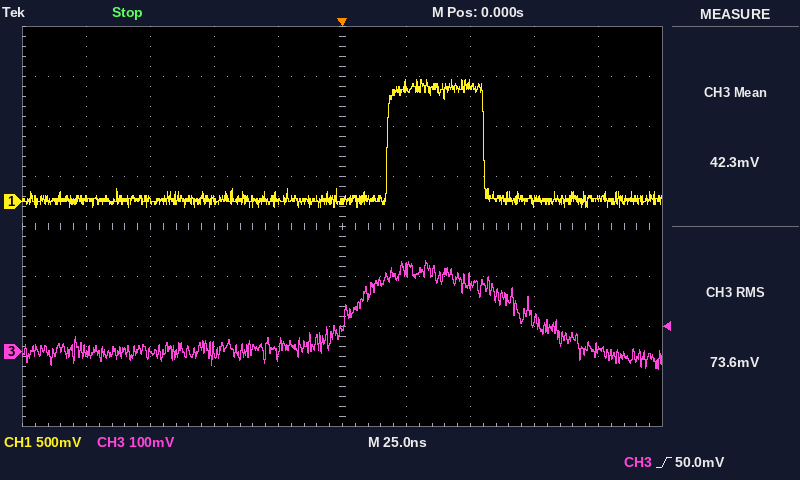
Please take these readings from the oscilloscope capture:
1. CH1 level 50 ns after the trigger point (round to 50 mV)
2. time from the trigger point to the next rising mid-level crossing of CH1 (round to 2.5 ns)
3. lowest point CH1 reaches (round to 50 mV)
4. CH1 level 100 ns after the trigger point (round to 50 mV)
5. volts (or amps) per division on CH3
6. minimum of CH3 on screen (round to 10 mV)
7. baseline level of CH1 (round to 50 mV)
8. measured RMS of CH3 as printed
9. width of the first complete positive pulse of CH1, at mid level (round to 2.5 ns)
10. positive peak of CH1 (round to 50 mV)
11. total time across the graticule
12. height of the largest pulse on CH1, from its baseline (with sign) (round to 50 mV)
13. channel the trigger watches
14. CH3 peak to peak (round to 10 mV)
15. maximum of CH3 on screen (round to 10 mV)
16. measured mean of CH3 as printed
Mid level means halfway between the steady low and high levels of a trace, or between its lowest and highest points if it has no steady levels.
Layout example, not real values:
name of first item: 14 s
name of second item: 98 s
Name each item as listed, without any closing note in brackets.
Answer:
CH1 level 50 ns after the trigger point: 1.15 V
time from the trigger point to the next rising mid-level crossing of CH1: 17.5 ns
lowest point CH1 reaches: -50 mV
CH1 level 100 ns after the trigger point: 50 mV
volts (or amps) per division on CH3: 100 mV
minimum of CH3 on screen: -40 mV
baseline level of CH1: 0 mV
measured RMS of CH3 as printed: 73.6 mV
width of the first complete positive pulse of CH1, at mid level: 37.5 ns
positive peak of CH1: 1.20 V
total time across the graticule: 250 ns
height of the largest pulse on CH1, from its baseline (with sign): +1.20 V
channel the trigger watches: CH3
CH3 peak to peak: 220 mV
maximum of CH3 on screen: 180 mV
measured mean of CH3 as printed: 42.3 mV
